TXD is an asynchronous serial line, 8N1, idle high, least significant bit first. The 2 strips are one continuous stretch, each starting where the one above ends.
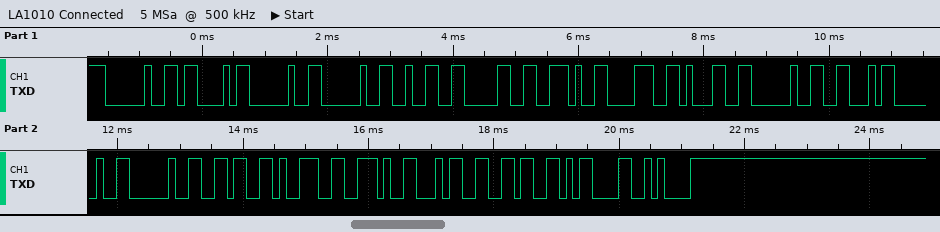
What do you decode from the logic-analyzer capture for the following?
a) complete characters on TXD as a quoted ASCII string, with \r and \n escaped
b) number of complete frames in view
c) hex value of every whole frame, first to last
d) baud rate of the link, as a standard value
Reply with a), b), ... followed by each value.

a) " C  20.81 F  69.46\r\n"
b) 20
c) 20 43 20 20 32 30 2E 38 31 20 46 20 20 36 39 2E 34 36 0D 0A
d) 9600 baud
